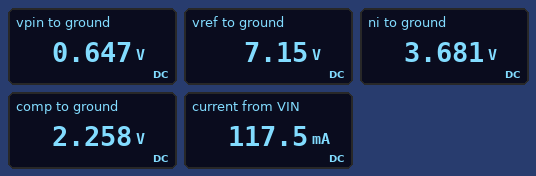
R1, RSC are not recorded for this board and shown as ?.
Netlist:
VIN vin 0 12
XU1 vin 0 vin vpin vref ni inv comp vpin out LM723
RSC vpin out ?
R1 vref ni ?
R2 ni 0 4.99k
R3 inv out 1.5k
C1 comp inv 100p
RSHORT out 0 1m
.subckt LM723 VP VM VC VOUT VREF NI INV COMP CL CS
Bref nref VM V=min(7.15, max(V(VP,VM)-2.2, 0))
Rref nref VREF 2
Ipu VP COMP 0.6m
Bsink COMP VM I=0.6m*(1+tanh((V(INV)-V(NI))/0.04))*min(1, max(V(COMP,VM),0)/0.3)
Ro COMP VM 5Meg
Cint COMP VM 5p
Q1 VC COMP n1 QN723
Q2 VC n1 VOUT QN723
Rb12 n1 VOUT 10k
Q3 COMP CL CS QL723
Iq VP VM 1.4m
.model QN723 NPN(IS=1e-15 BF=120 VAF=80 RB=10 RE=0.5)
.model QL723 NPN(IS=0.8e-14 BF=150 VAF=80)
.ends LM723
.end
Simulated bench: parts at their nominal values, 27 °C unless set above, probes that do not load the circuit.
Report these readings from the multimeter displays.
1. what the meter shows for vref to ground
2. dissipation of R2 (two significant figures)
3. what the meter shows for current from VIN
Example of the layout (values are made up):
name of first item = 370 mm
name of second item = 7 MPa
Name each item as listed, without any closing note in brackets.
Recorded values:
what the meter shows for vref to ground = 7.15 V
dissipation of R2 = 2.7 mW
what the meter shows for current from VIN = 117.5 mA
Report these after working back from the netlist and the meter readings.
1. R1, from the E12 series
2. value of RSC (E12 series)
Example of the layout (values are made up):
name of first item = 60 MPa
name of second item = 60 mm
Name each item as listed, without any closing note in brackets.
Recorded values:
R1, from the E12 series = 4.7 kΩ
value of RSC = 5.6 Ω
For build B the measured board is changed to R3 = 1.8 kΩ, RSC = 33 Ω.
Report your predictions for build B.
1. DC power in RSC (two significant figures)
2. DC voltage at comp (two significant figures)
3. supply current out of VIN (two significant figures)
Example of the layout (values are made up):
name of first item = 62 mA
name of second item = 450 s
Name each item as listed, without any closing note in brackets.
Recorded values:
DC power in RSC = 13 mW
DC voltage at comp = 2.1 V
supply current out of VIN = 22 mA
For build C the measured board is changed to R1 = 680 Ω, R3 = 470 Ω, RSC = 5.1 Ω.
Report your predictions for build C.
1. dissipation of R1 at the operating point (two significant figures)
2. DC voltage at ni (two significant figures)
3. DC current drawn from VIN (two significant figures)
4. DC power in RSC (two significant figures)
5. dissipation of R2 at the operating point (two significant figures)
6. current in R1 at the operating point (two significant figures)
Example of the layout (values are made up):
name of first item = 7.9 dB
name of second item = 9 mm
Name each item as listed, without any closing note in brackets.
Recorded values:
dissipation of R1 at the operating point = 1.1 mW
DC voltage at ni = 6.3 V
DC current drawn from VIN = 130 mA
DC power in RSC = 82 mW
dissipation of R2 at the operating point = 7.9 mW
current in R1 at the operating point = 1.3 mA
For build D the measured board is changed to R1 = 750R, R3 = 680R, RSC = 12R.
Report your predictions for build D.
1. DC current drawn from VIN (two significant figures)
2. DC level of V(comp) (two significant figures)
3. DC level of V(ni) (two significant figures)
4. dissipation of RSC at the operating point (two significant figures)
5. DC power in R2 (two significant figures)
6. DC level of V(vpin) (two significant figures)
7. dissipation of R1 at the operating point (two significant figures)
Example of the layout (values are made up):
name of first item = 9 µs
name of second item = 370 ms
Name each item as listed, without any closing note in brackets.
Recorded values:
DC current drawn from VIN = 56 mA
DC level of V(comp) = 2.2 V
DC level of V(ni) = 6.2 V
dissipation of RSC at the operating point = 35 mW
DC power in R2 = 7.7 mW
DC level of V(vpin) = 650 mV
dissipation of R1 at the operating point = 1.2 mW
